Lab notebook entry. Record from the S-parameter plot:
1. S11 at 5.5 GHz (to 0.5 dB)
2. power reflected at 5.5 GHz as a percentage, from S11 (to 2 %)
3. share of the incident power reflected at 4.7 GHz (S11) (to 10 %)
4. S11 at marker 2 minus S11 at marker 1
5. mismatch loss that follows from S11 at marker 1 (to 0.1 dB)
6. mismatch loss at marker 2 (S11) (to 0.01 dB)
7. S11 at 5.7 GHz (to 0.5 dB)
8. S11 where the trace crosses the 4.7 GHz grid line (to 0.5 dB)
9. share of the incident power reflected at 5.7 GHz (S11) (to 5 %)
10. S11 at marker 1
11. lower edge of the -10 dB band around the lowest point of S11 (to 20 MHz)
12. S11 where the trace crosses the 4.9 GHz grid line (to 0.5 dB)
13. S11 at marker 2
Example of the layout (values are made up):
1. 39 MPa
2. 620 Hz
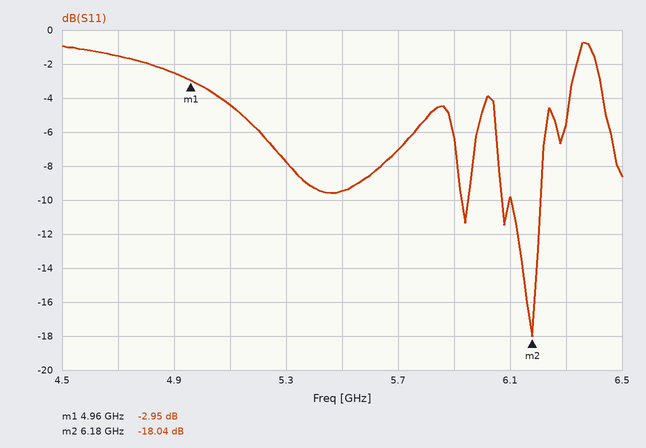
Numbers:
1. -9.5 dB
2. 12 %
3. 70 %
4. -15.09 dB
5. 3.1 dB
6. 0.07 dB
7. -7.0 dB
8. -1.5 dB
9. 20 %
10. -2.95 dB
11. 6.10 GHz
12. -2.5 dB
13. -18.04 dB
